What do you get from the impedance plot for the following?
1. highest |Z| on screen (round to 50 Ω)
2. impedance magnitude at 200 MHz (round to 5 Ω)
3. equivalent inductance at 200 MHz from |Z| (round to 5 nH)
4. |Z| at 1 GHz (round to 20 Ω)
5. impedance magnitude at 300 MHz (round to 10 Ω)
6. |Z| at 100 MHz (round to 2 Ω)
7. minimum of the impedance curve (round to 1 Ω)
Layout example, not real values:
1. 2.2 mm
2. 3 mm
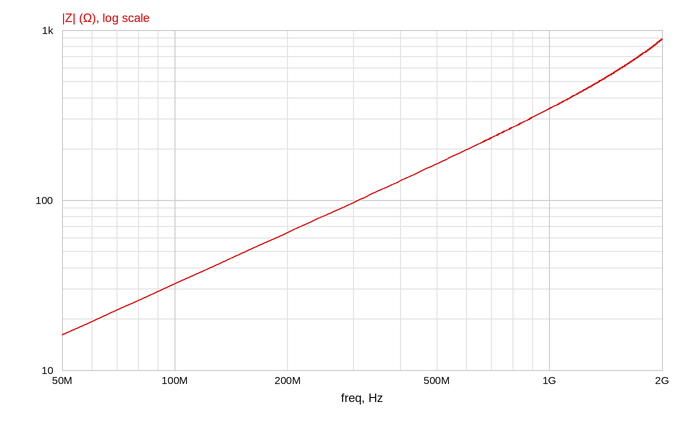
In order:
1. 900 Ω
2. 65 Ω
3. 50 nH
4. 340 Ω
5. 100 Ω
6. 32 Ω
7. 16 Ω
